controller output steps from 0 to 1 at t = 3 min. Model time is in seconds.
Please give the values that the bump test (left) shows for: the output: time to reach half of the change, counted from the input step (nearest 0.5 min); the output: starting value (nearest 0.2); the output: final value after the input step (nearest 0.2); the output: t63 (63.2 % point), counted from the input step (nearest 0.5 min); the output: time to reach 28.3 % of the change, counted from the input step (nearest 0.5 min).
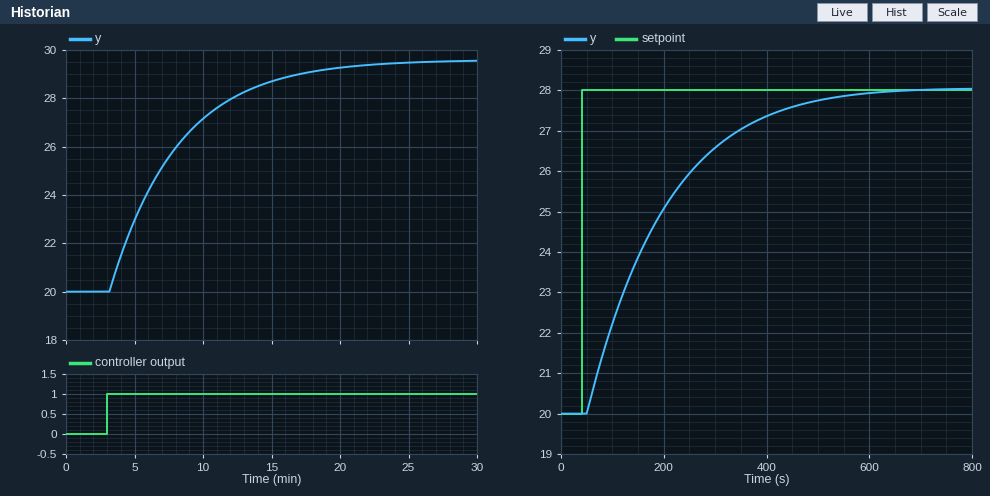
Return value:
3.5 min
20.0
29.6
5.0 min
2.0 min
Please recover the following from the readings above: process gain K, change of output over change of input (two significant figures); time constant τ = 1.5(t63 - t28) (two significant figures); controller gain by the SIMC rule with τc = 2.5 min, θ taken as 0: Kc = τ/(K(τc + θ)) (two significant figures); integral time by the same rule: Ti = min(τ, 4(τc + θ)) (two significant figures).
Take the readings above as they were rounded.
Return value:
9.6
4.5 min
0.19
4.5 min
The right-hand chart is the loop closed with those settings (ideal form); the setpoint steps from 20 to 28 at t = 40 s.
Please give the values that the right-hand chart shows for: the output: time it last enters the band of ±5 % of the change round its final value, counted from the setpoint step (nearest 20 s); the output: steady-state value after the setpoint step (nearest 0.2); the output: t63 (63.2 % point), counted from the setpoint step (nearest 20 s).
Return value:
420 s
28.0
160 s
